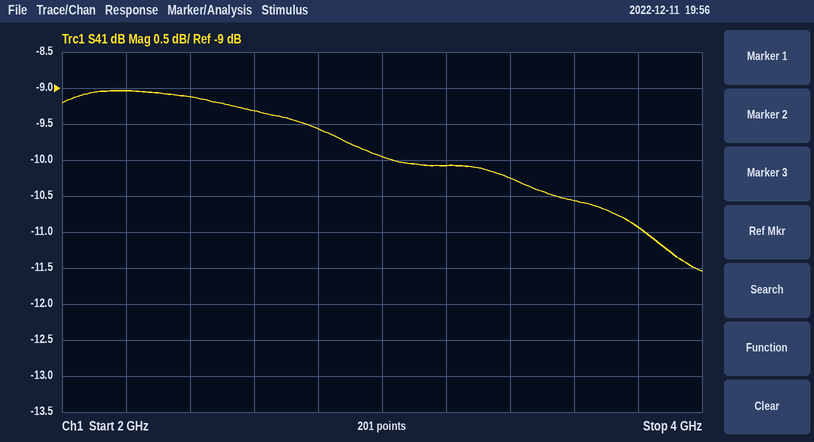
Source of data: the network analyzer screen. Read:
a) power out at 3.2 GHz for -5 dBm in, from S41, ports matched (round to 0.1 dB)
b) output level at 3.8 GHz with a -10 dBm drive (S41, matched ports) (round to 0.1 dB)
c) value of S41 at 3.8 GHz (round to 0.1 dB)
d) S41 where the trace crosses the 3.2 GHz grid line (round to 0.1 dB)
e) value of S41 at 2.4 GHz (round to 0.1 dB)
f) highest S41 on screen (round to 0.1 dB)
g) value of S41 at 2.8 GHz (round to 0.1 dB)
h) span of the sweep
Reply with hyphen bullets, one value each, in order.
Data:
- -15.1 dBm
- -20.9 dBm
- -10.9 dB
- -10.1 dB
- -9.1 dB
- -9.0 dB
- -9.6 dB
- 2 GHz
